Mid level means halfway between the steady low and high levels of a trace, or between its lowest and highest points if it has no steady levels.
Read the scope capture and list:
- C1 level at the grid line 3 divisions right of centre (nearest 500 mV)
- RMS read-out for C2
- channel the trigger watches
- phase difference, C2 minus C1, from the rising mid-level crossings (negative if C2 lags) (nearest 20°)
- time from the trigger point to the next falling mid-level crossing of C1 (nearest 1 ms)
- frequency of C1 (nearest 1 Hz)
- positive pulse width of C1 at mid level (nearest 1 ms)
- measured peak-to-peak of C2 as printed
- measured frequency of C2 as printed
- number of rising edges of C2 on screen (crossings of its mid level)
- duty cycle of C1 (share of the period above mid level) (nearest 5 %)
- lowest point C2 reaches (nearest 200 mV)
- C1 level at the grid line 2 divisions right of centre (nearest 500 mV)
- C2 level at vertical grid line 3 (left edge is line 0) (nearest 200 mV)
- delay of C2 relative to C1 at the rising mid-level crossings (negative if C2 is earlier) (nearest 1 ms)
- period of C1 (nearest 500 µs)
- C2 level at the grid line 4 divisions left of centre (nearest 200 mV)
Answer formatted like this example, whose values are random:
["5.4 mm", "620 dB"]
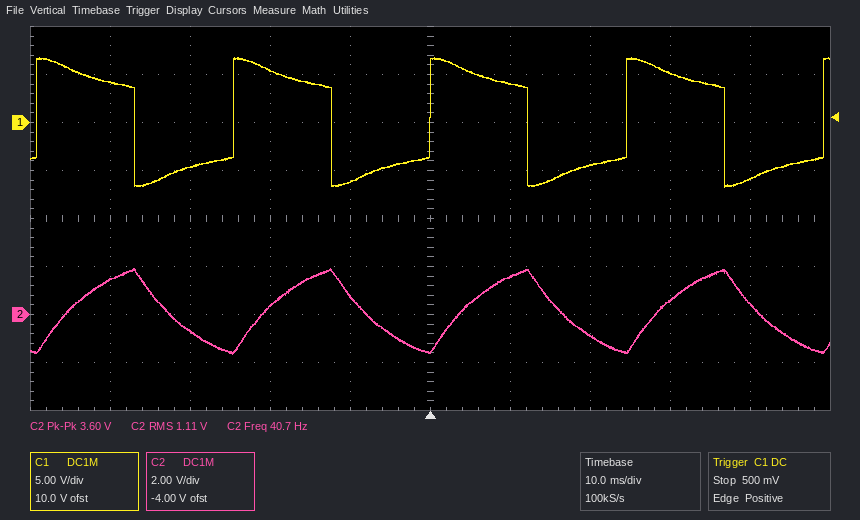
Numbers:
["5.0 V", "1.11 V", "C1", "-60°", "12 ms", "41 Hz", "12 ms", "3.60 V", "40.7 Hz", "4", "50 %", "-1.6 V", "-4.5 V", "400 mV", "+4 ms", "24.5 ms", "1.4 V"]
